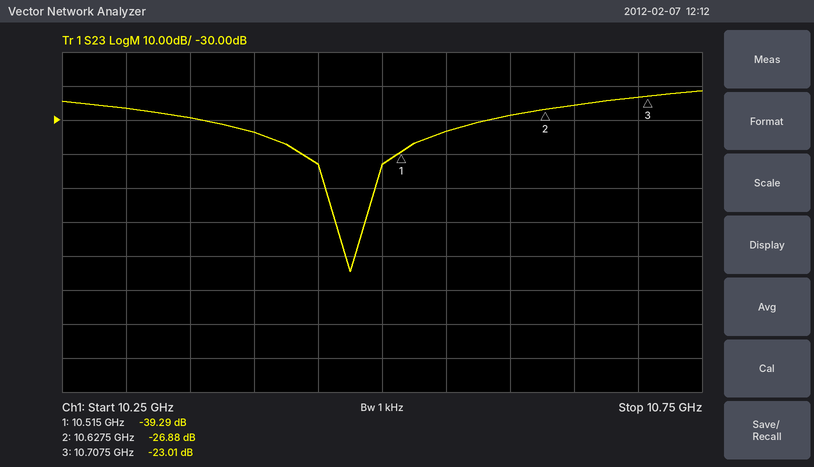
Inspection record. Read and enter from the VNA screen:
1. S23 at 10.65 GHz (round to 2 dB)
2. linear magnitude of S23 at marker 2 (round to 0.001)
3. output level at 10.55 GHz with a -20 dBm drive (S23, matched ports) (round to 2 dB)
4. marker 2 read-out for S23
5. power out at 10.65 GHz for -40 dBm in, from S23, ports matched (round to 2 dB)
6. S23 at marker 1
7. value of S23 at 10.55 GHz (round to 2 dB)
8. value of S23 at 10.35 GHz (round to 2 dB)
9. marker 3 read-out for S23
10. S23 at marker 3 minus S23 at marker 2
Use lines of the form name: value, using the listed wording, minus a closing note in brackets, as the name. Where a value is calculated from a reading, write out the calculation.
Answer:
S23 at 10.65 GHz: -26 dB
linear magnitude of S23 at marker 2: 10^(-26.88/20) ≈ 0.045
output level at 10.55 GHz with a -20 dBm drive (S23, matched ports): -20 dBm + (-34 dB) = -54 dBm
marker 2 read-out for S23: -26.88 dB
power out at 10.65 GHz for -40 dBm in, from S23, ports matched: -40 dBm + (-26 dB) = -66 dBm
S23 at marker 1: -39.29 dB
value of S23 at 10.55 GHz: -34 dB
value of S23 at 10.35 GHz: -30 dB
marker 3 read-out for S23: -23.01 dB
S23 at marker 3 minus S23 at marker 2: -23.01 − (-26.88) = 3.87 dB
